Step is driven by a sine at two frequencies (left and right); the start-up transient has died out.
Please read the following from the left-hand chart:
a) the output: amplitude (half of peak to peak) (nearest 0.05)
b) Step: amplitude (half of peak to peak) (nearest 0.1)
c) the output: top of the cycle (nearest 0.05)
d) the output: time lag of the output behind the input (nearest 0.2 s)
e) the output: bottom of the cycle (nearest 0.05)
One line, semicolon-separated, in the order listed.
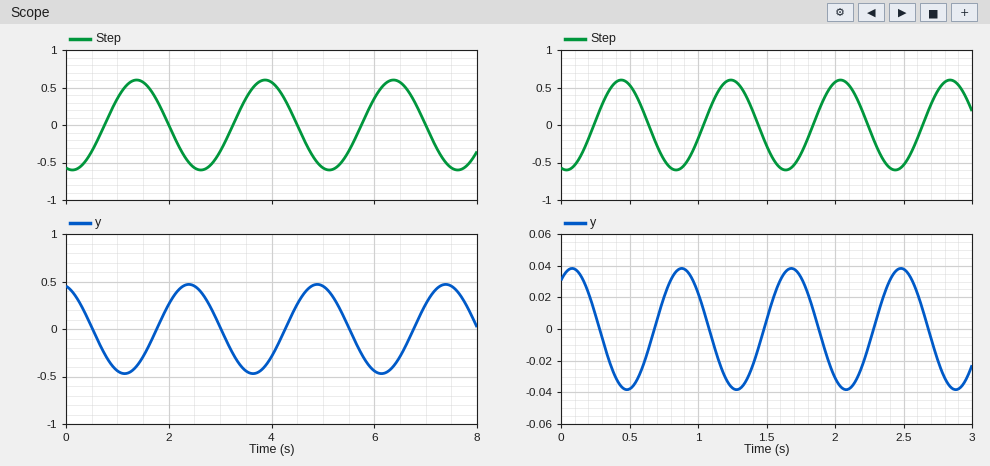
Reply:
0.45; 0.6; 0.45; 1.0 s; -0.45
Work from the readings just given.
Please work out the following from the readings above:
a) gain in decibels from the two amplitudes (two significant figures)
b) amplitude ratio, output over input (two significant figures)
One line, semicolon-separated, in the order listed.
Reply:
-2.5 dB; 0.75
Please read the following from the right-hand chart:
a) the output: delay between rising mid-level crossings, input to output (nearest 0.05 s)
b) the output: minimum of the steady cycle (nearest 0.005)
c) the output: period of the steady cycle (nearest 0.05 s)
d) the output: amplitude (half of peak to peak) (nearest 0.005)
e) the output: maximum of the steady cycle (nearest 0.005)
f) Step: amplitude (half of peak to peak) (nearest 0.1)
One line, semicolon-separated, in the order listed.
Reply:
0.45 s; -0.040; 0.80 s; 0.040; 0.040; 0.6
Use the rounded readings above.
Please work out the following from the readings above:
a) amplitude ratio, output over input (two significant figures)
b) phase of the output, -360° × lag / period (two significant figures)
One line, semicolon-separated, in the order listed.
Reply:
0.067; -200°
